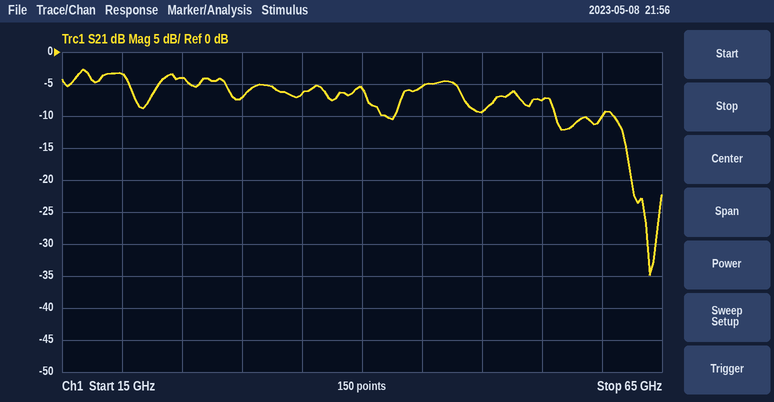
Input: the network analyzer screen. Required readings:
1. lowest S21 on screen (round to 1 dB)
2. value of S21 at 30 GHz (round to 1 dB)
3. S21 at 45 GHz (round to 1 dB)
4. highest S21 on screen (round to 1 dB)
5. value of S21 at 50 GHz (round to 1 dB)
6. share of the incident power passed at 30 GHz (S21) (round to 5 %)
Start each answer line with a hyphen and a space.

- -35 dB
- -7 dB
- -5 dB
- -3 dB
- -9 dB
- 20 %
